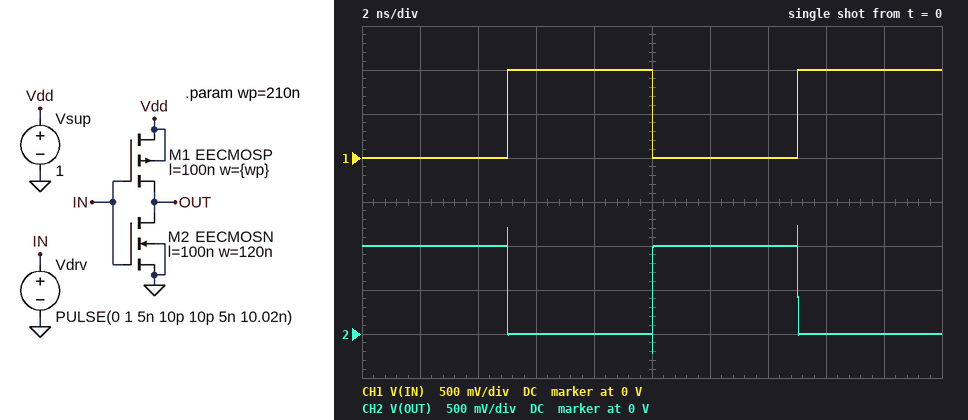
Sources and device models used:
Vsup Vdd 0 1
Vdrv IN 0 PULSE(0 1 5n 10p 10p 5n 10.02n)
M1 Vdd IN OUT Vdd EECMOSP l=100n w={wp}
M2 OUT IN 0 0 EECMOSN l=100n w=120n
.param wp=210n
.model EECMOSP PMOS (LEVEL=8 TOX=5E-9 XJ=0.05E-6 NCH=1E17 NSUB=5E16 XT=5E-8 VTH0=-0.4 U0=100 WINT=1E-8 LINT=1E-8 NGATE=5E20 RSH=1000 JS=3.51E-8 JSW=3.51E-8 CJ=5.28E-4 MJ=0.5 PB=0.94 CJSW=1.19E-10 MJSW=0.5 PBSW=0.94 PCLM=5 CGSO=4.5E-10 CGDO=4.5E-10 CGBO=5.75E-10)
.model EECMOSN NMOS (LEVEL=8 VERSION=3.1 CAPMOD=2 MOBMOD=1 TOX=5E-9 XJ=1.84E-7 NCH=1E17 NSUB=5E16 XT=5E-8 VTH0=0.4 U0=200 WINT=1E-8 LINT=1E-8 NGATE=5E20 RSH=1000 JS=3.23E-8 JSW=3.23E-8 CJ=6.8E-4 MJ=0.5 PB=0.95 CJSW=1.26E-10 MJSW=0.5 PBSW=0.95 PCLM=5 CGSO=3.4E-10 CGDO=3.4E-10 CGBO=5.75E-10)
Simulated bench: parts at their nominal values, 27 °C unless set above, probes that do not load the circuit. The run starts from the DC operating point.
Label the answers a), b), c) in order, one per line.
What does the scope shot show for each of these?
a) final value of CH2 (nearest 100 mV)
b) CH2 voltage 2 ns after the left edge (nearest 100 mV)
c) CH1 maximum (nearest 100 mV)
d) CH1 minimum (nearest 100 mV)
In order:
a) 0 V
b) 1.0 V
c) 1.0 V
d) 0 V
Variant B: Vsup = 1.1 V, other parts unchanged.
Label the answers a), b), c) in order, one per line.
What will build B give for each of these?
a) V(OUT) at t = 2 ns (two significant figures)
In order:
a) 1.1 V
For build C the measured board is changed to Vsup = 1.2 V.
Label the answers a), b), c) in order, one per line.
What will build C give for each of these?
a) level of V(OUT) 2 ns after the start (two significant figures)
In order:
a) 1.2 V
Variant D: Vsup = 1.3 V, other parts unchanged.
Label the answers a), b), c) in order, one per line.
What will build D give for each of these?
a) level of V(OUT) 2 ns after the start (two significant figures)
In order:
a) 1.3 V
